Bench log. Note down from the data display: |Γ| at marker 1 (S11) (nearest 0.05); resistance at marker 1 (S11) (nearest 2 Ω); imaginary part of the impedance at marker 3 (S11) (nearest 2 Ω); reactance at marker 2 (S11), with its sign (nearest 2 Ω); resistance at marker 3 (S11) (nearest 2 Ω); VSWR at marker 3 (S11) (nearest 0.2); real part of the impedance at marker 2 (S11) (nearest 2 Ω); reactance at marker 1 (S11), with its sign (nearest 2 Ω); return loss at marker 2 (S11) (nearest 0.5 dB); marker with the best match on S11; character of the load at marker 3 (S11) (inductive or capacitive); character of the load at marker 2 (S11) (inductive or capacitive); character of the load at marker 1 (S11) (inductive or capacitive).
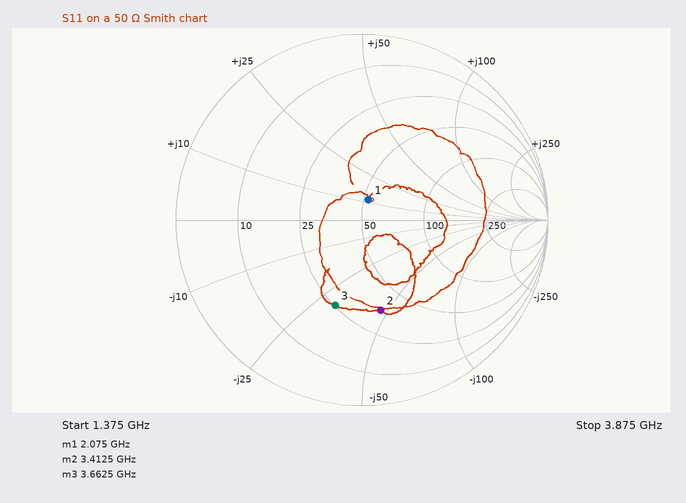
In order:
0.10
52 Ω
-30 Ω
-46 Ω
26 Ω
2.8
36 Ω
+12 Ω
6.0 dB
marker 1
capacitive
capacitive
inductive
